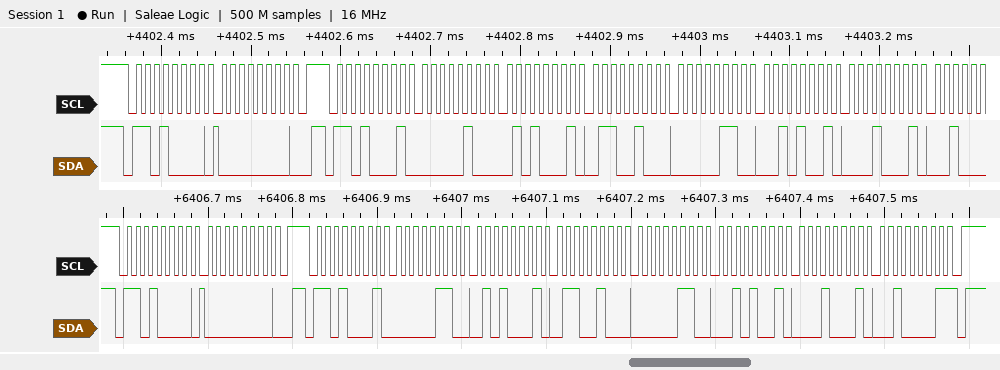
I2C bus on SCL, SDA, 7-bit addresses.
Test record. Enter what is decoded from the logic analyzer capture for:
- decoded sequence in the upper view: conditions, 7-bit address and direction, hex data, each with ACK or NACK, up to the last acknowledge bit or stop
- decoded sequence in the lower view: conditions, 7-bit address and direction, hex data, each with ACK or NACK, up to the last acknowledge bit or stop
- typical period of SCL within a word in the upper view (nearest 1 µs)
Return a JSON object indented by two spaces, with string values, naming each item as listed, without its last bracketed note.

{
  "decoded sequence in the upper view: conditions, 7-bit address and direction, hex data, each with ACK or NACK, up to the last acknowledge bit or stop": "start, address 68 write ACK, 00 ACK, stop, start, address 68 read ACK, 04 ACK, 51 ACK, 64 ACK, 06 ACK, 29 ACK, 11 ACK",
  "decoded sequence in the lower view: conditions, 7-bit address and direction, hex data, each with ACK or NACK, up to the last acknowledge bit or stop": "start, address 68 write ACK, 00 ACK, stop, start, address 68 read ACK, 06 ACK, 51 ACK, 64 ACK, 06 ACK, 29 ACK, 11 ACK, 21 NACK, stop",
  "typical period of SCL within a word in the upper view": "10 µs"
}
